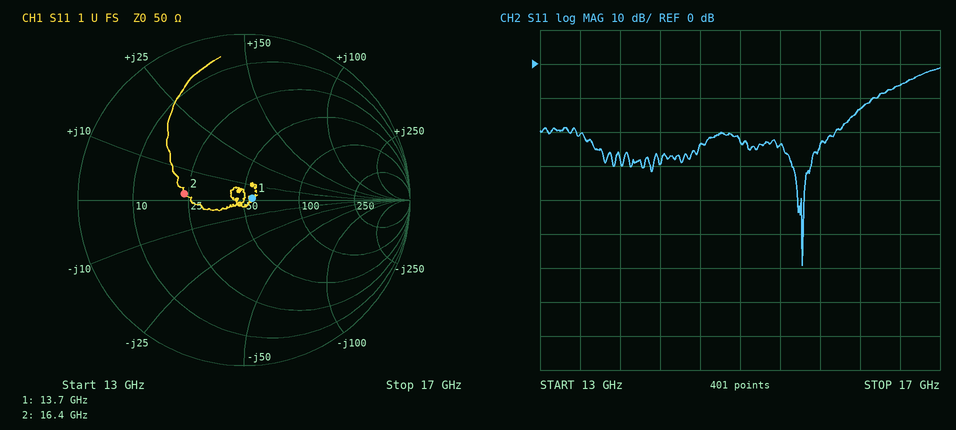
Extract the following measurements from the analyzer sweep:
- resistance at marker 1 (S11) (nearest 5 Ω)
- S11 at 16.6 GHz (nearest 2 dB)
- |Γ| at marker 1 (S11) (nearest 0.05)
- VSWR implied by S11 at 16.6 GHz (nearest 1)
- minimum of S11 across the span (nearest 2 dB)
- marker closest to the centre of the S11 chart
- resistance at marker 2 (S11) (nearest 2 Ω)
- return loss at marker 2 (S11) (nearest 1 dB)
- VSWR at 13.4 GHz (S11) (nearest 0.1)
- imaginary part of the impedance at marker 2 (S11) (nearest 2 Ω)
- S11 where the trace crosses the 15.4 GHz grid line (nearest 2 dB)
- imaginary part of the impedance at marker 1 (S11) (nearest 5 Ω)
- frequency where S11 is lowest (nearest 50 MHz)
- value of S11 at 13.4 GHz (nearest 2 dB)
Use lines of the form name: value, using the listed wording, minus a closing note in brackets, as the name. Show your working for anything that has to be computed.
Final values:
resistance at marker 1 (S11): 55 Ω
S11 at 16.6 GHz: -6 dB
|Γ| at marker 1 (S11): 0.05
VSWR implied by S11 at 16.6 GHz: |Γ| = 10^(-6/20) = 0.5012; VSWR = (1 + 0.5012)/(1 − 0.5012) ≈ 3
minimum of S11 across the span: -60 dB
marker closest to the centre of the S11 chart: marker 1
resistance at marker 2 (S11): 24 Ω
return loss at marker 2 (S11): 9 dB
VSWR at 13.4 GHz (S11): |Γ| = 10^(-20/20) = 0.1000; VSWR = (1 + 0.1000)/(1 − 0.1000) ≈ 1.2
imaginary part of the impedance at marker 2 (S11): +2 Ω
S11 where the trace crosses the 15.4 GHz grid line: -24 dB
imaginary part of the impedance at marker 1 (S11): 0 Ω
frequency where S11 is lowest: 15.60 GHz
value of S11 at 13.4 GHz: -20 dB
